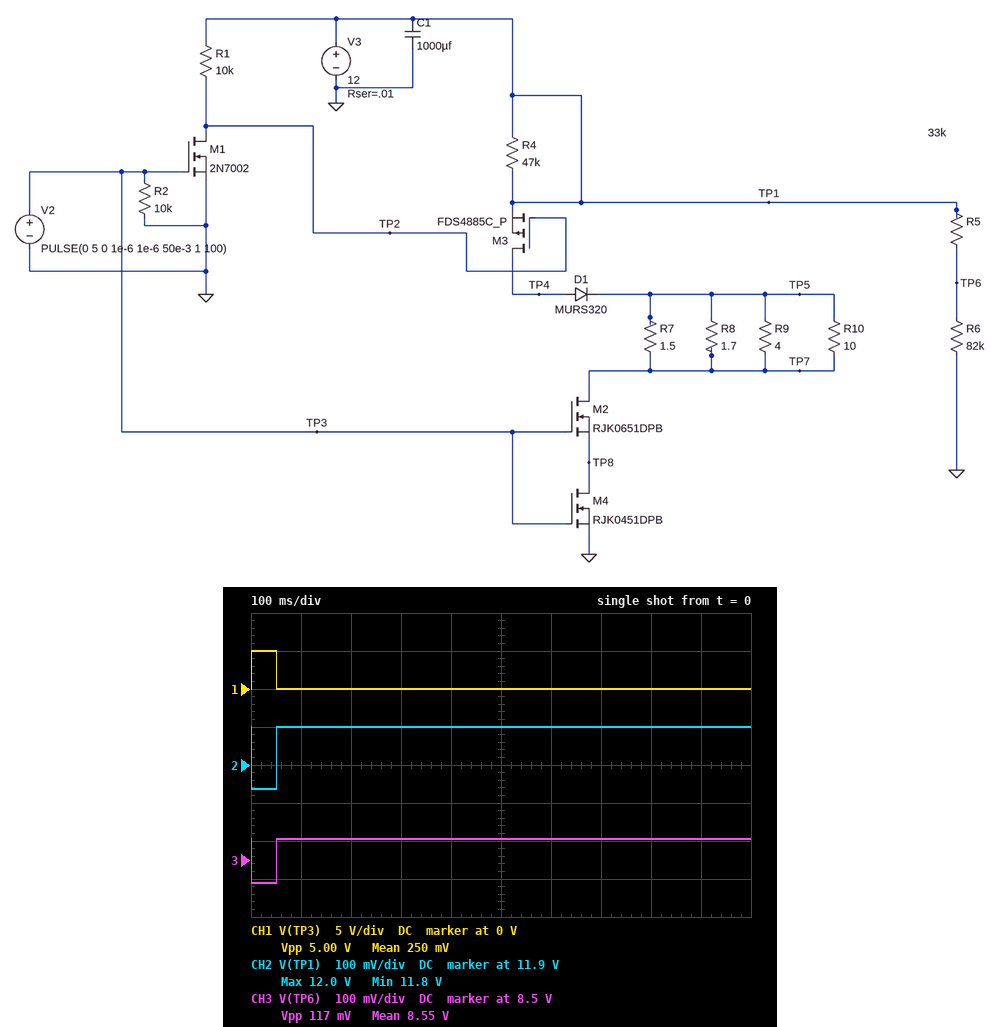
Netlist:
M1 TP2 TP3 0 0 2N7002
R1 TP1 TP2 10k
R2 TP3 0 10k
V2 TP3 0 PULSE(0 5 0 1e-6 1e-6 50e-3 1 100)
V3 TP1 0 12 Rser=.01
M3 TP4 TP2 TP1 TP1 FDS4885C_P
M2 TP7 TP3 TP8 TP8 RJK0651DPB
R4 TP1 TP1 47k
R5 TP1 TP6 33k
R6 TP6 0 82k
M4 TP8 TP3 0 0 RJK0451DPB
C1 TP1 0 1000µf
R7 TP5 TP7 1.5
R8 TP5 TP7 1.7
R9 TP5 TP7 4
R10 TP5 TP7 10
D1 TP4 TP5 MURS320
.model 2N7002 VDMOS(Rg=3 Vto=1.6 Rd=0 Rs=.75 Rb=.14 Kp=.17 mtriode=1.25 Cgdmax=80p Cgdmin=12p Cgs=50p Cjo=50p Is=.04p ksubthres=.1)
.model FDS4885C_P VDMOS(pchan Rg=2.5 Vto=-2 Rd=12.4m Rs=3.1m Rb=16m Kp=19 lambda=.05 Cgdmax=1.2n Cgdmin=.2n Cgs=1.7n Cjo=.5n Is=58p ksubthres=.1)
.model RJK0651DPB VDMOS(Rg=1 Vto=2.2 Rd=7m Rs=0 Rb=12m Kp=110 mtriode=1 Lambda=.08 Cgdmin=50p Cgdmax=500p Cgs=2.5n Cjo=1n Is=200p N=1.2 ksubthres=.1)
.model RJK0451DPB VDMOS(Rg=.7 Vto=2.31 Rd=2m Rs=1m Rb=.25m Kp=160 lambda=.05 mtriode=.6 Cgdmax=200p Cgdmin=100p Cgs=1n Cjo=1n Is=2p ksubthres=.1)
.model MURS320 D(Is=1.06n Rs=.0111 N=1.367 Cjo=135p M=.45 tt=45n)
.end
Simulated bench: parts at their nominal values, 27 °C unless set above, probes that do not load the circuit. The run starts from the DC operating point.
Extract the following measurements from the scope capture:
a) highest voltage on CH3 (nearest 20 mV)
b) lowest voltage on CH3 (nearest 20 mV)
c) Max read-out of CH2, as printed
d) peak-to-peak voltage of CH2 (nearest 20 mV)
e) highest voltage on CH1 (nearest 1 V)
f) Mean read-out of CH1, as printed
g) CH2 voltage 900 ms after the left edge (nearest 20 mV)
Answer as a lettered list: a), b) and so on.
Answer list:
a) 8.56 V
b) 8.44 V
c) 12.0 V
d) 160 mV
e) 5 V
f) 250 mV
g) 12.00 V
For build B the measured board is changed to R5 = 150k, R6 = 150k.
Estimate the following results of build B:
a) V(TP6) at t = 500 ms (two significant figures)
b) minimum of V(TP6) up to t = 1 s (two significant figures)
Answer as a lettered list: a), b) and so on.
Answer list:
a) 6.0 V
b) 5.9 V
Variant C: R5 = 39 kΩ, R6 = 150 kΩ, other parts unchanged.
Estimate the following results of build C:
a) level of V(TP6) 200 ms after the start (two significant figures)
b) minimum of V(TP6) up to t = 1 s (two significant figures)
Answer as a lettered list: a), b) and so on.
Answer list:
a) 9.5 V
b) 9.4 V
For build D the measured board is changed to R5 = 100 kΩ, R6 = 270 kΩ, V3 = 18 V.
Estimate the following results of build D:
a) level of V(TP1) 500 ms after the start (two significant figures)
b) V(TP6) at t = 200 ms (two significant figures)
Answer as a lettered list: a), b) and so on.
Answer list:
a) 18 V
b) 13 V
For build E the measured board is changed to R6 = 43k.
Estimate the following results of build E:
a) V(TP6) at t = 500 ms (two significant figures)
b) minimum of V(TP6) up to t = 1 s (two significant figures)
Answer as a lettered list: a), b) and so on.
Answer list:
a) 6.8 V
b) 6.7 V
